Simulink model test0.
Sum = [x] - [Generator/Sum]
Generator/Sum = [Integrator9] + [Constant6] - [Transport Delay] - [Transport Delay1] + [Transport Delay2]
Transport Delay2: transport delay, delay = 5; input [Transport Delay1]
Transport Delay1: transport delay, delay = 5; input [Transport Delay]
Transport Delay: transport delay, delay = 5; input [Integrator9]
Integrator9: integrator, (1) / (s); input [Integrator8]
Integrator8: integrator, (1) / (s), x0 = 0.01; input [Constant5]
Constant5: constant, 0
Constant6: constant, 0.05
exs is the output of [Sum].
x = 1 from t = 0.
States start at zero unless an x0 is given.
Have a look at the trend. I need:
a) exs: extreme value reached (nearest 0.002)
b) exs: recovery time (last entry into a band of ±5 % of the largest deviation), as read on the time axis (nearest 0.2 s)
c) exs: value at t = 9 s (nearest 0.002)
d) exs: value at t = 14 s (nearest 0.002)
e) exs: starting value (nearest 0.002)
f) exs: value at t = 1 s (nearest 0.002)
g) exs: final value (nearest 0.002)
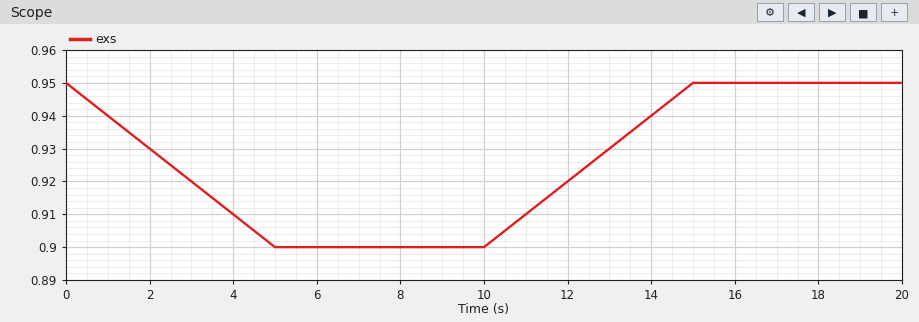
0.900
14.8 s
0.900
0.940
0.950
0.940
0.950
